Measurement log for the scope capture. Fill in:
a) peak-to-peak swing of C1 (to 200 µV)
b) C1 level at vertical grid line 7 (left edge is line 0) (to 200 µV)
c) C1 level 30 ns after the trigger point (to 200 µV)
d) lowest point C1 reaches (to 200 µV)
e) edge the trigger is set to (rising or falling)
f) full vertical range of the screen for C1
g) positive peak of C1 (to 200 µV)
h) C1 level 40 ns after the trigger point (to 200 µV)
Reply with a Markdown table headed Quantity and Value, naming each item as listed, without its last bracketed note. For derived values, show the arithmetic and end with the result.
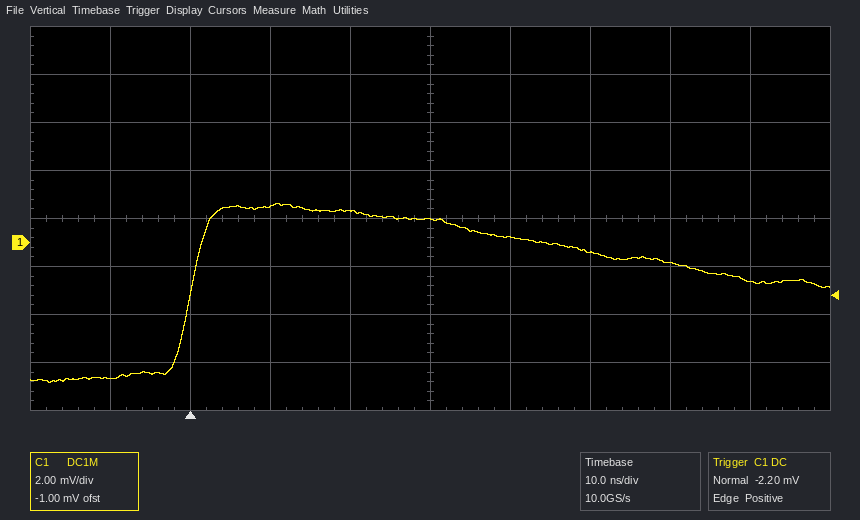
| Quantity | Value |
|---|---|
| peak-to-peak swing of C1 | 1.6 mV − (-5.8 mV) = 7.4 mV |
| C1 level at vertical grid line 7 (left edge is line 0) | -400 µV |
| C1 level 30 ns after the trigger point | 1.0 mV |
| lowest point C1 reaches | -5.8 mV |
| edge the trigger is set to | rising |
| full vertical range of the screen for C1 | 16 mV |
| positive peak of C1 | 1.6 mV |
| C1 level 40 ns after the trigger point | 200 µV |
